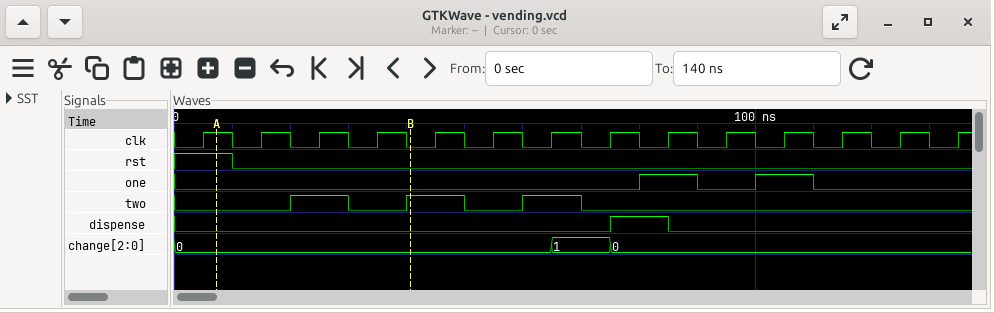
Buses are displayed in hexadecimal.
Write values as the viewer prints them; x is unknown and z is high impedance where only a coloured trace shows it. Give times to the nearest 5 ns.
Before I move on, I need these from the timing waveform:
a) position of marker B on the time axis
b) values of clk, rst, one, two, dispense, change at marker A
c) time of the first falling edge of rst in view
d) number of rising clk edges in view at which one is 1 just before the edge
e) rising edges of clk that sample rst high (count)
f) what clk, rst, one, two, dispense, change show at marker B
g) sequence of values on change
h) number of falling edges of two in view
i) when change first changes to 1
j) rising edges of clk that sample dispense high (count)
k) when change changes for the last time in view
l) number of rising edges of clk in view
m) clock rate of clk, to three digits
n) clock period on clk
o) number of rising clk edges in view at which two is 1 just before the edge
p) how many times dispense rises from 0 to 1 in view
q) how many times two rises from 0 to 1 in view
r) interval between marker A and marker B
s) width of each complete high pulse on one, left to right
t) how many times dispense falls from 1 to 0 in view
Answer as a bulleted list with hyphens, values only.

- 40 ns
- clk=1, rst=1, one=0, two=0, dispense=0, change=0
- 10 ns
- 2
- 1
- clk=0, rst=0, one=0, two=1, dispense=0, change=0
- 0, 1, 0
- 3
- 65 ns
- 1
- 75 ns
- 14
- 100 MHz
- 10 ns
- 3
- 1
- 3
- 35 ns
- 10 ns, 10 ns
- 1
